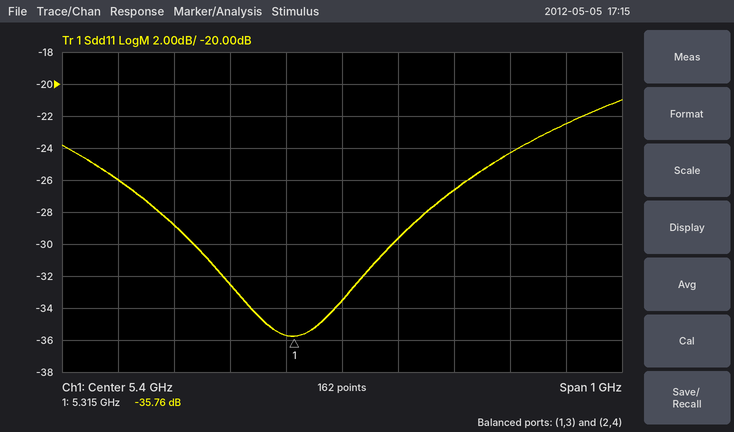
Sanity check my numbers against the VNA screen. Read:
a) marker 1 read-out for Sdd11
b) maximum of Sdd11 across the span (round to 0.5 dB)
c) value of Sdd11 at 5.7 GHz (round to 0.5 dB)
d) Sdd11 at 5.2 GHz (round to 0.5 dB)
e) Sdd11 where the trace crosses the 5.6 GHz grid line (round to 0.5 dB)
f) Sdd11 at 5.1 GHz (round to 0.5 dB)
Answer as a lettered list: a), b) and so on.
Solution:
a) -35.76 dB
b) -21.0 dB
c) -24.5 dB
d) -32.5 dB
e) -26.5 dB
f) -29.0 dB
